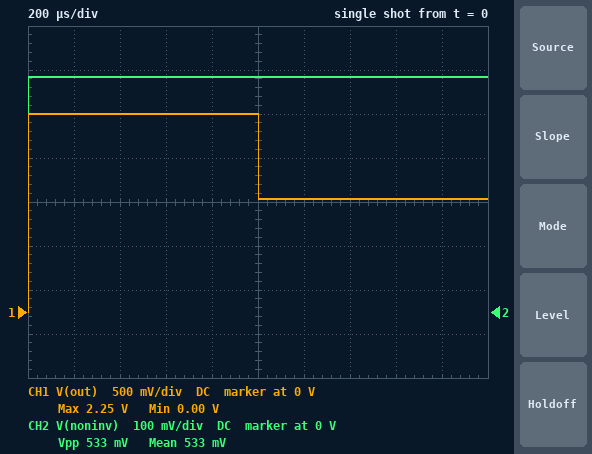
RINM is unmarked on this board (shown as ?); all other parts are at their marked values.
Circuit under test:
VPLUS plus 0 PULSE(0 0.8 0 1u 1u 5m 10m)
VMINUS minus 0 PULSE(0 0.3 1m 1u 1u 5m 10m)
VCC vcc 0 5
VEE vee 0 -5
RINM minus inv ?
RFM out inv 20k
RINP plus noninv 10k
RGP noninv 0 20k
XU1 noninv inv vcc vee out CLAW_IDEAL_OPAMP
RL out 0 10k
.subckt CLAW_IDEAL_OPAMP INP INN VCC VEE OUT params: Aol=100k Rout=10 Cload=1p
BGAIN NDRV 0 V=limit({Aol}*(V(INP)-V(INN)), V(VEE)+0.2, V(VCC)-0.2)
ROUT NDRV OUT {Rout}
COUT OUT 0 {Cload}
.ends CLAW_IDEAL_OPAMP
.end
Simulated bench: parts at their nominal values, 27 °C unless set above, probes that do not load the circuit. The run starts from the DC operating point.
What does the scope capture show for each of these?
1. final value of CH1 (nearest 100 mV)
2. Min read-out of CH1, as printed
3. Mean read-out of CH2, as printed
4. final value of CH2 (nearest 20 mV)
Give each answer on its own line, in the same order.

1.3 V
0.00 V
533 mV
540 mV
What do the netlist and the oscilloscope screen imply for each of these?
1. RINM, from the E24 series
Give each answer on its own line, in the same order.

6.2 kΩ
